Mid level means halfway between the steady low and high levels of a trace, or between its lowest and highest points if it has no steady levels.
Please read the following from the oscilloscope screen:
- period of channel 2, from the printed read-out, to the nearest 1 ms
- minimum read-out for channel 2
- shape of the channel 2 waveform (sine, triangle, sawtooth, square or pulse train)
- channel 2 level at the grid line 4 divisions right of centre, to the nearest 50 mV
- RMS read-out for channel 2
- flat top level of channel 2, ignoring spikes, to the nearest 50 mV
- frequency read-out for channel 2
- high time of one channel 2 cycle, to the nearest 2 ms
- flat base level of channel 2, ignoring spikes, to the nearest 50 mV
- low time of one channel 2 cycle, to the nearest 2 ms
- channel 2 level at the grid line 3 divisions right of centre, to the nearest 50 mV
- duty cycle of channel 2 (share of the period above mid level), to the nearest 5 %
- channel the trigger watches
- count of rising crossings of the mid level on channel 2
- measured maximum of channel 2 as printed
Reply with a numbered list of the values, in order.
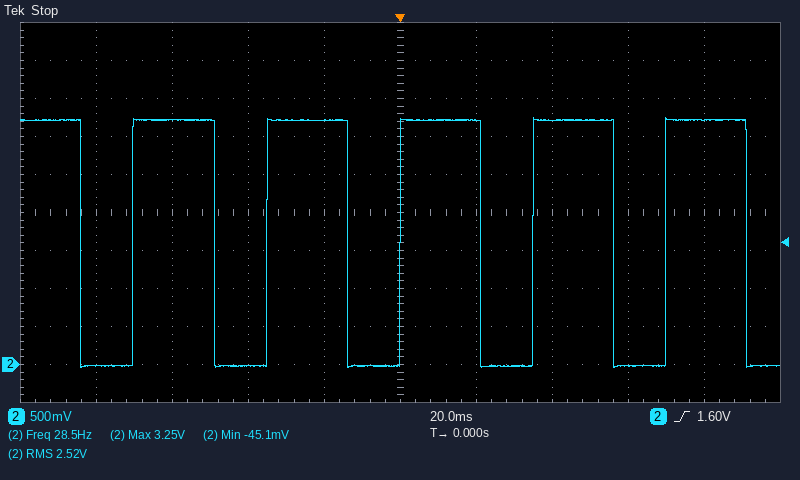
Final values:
1. 35 ms
2. -45.1 mV
3. pulse train
4. 3.20 V
5. 2.52 V
6. 3.20 V
7. 28.5 Hz
8. 22 ms
9. 0 mV
10. 14 ms
11. 0 mV
12. 60 %
13. channel 2
14. 5
15. 3.25 V
